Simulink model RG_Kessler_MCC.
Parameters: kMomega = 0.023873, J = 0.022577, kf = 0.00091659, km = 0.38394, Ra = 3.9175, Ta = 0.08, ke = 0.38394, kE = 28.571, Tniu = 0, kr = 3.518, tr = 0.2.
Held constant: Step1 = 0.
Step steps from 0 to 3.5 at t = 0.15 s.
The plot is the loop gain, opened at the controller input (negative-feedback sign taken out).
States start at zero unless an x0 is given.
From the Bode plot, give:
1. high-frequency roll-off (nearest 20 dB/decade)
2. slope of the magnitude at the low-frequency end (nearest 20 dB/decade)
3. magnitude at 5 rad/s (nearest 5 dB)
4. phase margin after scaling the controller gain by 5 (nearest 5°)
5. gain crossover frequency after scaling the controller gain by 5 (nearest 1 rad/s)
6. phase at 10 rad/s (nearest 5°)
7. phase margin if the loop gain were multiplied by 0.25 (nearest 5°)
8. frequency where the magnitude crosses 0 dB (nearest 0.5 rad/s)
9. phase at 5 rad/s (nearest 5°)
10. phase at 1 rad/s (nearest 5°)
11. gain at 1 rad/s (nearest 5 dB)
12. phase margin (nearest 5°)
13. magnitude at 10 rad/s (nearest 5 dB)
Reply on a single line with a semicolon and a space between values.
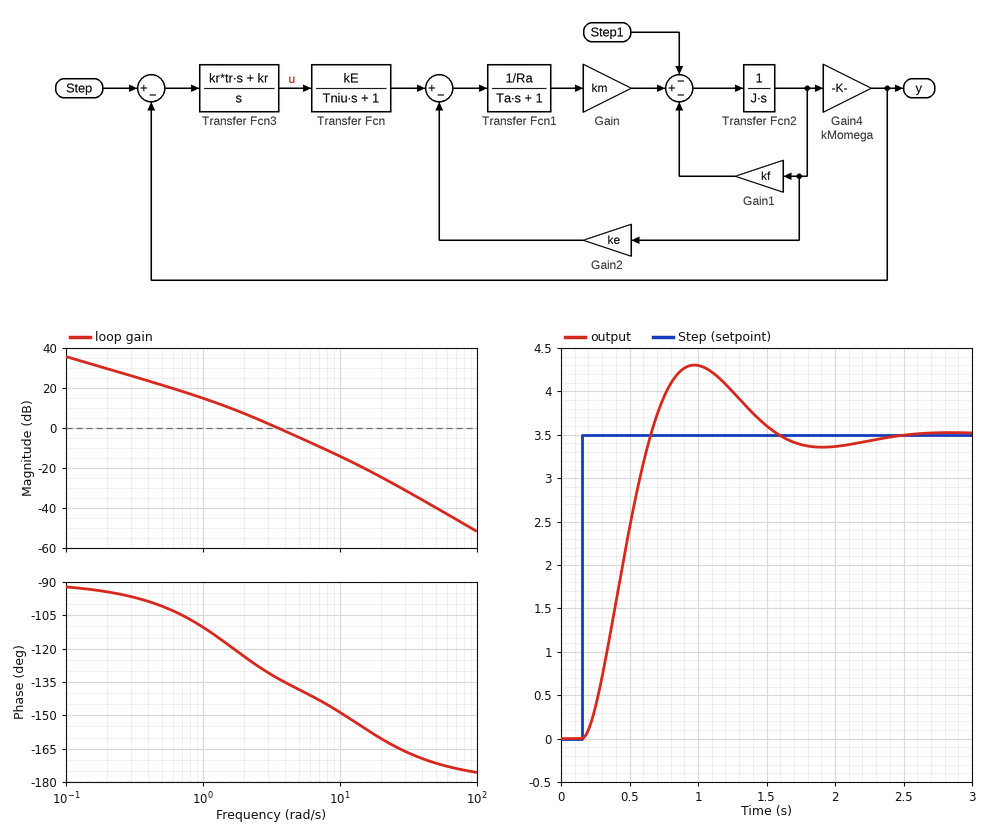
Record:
-40 dB/decade; -20 dB/decade; -5 dB; 30°; 10 rad/s; -150°; 65°; 3.5 rad/s; -140°; -110°; 15 dB; 45°; -15 dB
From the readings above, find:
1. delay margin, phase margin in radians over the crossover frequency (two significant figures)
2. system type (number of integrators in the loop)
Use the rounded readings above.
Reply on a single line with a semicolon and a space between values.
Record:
0.22 s; 1
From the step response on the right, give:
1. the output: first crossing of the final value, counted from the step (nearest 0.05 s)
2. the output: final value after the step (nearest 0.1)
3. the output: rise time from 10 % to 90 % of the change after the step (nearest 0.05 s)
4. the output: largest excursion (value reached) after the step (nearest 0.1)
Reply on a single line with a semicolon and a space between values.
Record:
0.50 s; 3.5; 0.35 s; 4.3
